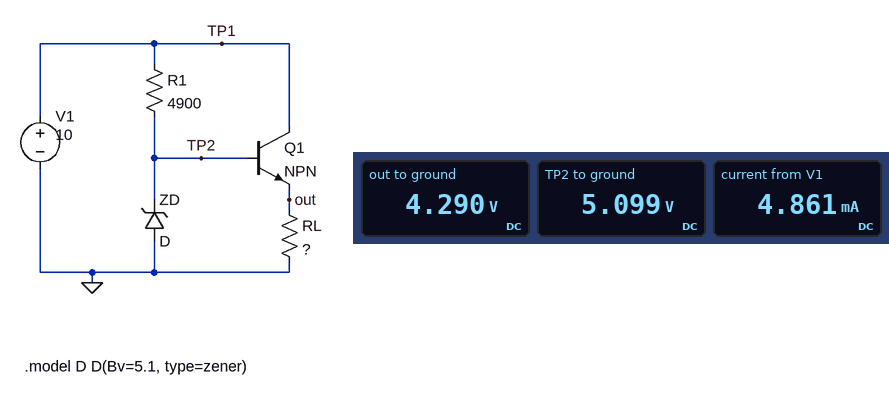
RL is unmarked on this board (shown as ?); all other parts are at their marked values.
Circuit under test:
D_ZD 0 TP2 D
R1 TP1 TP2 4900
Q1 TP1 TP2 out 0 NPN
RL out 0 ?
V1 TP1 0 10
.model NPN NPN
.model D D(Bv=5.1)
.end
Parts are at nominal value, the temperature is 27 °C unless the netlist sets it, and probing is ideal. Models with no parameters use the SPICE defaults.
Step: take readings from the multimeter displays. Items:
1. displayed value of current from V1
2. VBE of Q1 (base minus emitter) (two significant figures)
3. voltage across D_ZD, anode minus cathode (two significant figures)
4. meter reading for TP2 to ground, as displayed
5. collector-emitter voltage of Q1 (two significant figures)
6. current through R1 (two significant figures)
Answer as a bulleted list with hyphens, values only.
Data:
- 4.861 mA
- 810 mV
- -5.1 V
- 5.099 V
- 5.7 V
- 1.0 mA
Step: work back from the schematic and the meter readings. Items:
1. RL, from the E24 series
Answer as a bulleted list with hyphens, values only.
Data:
- 1.1 kΩ
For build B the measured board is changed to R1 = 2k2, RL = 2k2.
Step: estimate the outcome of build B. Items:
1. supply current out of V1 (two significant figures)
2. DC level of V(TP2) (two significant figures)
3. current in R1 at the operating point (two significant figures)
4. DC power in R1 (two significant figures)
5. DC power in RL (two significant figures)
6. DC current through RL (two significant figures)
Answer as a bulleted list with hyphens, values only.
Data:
- 4.2 mA
- 5.1 V
- 2.2 mA
- 11 mW
- 8.5 mW
- 2.0 mA
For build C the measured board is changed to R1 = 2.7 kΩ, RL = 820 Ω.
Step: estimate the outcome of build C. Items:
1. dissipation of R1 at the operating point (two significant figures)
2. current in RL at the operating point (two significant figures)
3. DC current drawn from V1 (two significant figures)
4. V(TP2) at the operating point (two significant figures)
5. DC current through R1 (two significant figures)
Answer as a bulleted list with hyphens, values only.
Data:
- 8.8 mW
- 5.2 mA
- 7.0 mA
- 5.1 V
- 1.8 mA
